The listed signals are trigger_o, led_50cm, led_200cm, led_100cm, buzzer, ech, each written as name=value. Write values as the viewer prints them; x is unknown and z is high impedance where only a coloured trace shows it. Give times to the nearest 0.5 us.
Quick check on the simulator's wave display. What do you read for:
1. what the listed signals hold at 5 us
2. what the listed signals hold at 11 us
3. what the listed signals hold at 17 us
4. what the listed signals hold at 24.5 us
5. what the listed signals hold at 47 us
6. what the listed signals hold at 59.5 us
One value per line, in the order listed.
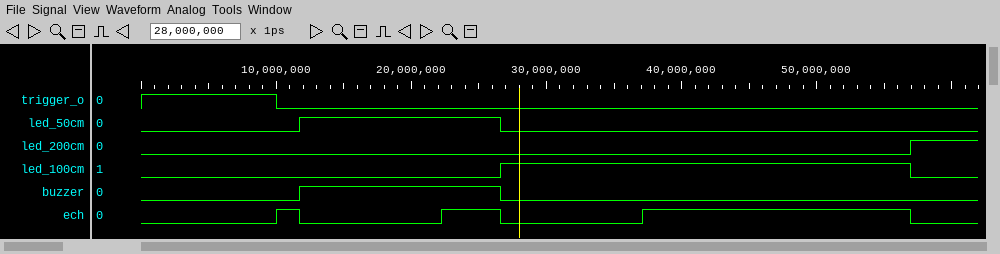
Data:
trigger_o=1, led_50cm=0, led_200cm=0, led_100cm=0, buzzer=0, ech=0
trigger_o=0, led_50cm=0, led_200cm=0, led_100cm=0, buzzer=0, ech=1
trigger_o=0, led_50cm=1, led_200cm=0, led_100cm=0, buzzer=1, ech=0
trigger_o=0, led_50cm=1, led_200cm=0, led_100cm=0, buzzer=1, ech=1
trigger_o=0, led_50cm=0, led_200cm=0, led_100cm=1, buzzer=0, ech=1
trigger_o=0, led_50cm=0, led_200cm=1, led_100cm=0, buzzer=0, ech=0
